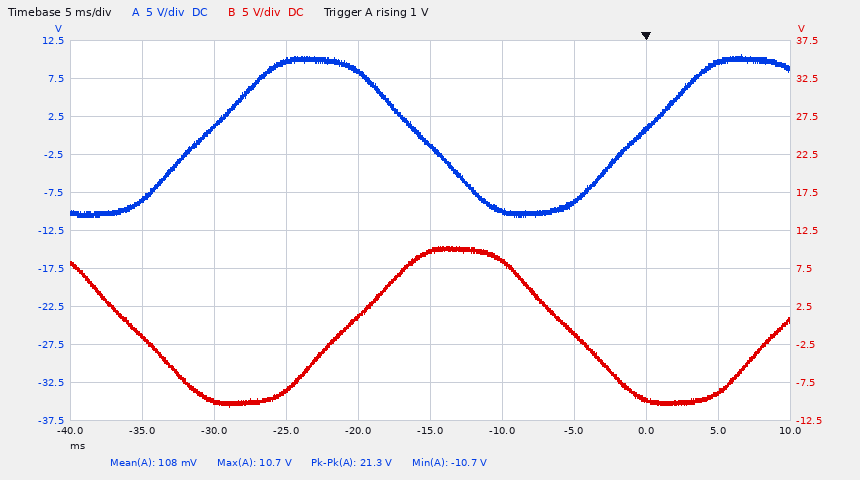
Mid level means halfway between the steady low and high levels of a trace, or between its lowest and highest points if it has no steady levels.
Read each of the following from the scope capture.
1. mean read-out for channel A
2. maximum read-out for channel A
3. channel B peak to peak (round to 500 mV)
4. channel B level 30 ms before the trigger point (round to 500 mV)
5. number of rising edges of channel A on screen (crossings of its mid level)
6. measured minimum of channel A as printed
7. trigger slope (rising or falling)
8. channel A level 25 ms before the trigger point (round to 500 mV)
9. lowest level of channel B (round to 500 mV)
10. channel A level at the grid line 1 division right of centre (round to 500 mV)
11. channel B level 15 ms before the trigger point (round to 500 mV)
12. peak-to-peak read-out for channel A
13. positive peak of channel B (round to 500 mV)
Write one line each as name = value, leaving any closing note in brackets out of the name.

mean read-out for channel A = 108 mV
maximum read-out for channel A = 10.7 V
channel B peak to peak = 21.0 V
channel B level 30 ms before the trigger point = -10.0 V
number of rising edges of channel A on screen = 2
measured minimum of channel A as printed = -10.7 V
trigger slope = rising
channel A level 25 ms before the trigger point = 10.0 V
lowest level of channel B = -10.5 V
channel A level at the grid line 1 division right of centre = -10.0 V
channel B level 15 ms before the trigger point = 10.0 V
peak-to-peak read-out for channel A = 21.3 V
positive peak of channel B = 10.5 V
